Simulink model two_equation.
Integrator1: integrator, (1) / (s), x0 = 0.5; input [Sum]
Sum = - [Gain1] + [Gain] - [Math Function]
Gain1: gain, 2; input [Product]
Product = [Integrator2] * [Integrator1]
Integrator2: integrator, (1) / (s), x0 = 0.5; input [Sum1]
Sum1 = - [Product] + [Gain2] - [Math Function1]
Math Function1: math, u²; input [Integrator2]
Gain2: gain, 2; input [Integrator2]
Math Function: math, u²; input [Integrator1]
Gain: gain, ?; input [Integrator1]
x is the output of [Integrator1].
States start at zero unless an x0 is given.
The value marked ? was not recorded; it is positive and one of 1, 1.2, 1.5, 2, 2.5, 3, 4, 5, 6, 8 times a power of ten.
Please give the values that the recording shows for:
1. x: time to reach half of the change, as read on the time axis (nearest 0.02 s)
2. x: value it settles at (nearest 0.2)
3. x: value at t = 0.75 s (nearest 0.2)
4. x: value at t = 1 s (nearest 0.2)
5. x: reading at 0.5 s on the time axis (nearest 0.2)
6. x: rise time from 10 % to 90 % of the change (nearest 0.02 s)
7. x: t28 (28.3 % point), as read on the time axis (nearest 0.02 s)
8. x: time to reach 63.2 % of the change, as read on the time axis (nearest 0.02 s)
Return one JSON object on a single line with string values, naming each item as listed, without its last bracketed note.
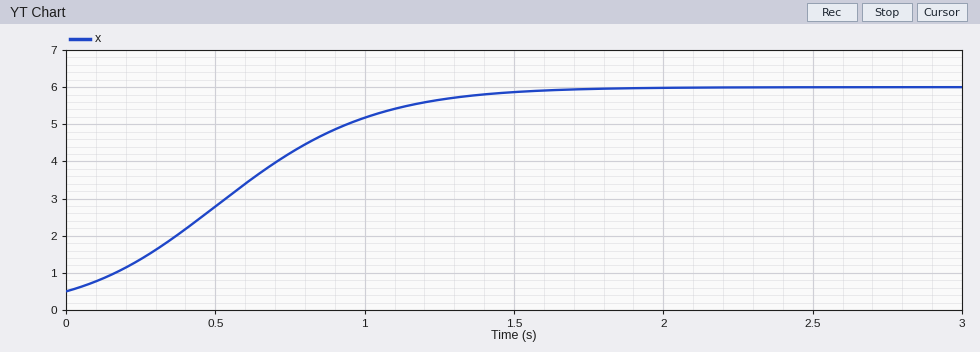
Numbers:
{"x: time to reach half of the change, as read on the time axis": "0.58 s", "x: value it settles at": "6.0", "x: value at t = 0.75 s": "4.2", "x: value at t = 1 s": "5.2", "x: reading at 0.5 s on the time axis": "2.8", "x: rise time from 10 % to 90 % of the change": "0.94 s", "x: t28 (28.3 % point), as read on the time axis": "0.38 s", "x: time to reach 63.2 % of the change, as read on the time axis": "0.70 s"}
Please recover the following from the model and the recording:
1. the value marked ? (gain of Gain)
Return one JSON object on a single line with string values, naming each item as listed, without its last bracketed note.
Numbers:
{"the value marked ?": "6"}
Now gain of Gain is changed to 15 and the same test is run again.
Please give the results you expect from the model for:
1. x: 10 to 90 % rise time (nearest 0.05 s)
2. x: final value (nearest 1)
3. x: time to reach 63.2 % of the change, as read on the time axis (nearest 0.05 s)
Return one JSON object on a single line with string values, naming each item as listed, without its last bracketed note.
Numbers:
{"x: 10 to 90 % rise time": "0.30 s", "x: final value": "15", "x: time to reach 63.2 % of the change, as read on the time axis": "0.30 s"}
